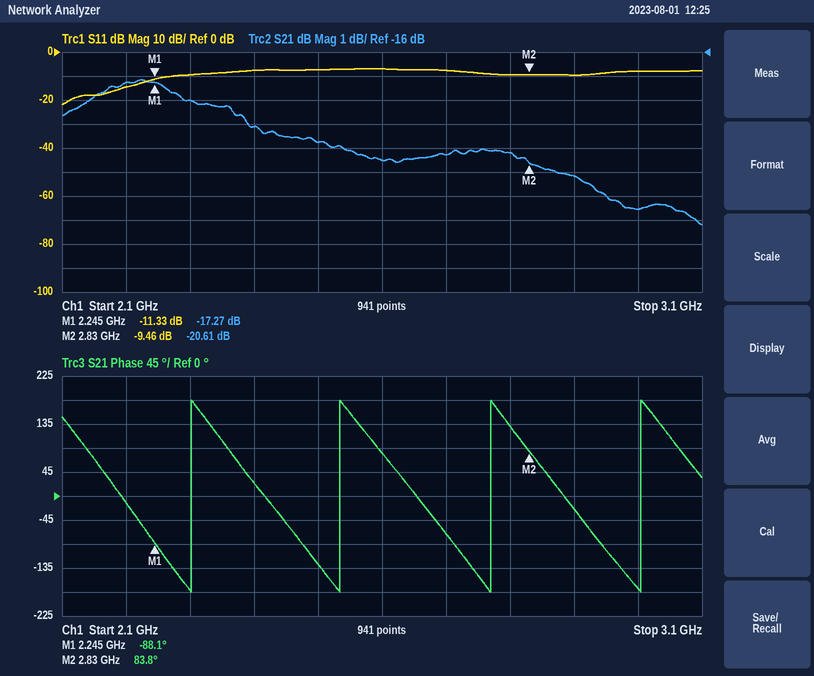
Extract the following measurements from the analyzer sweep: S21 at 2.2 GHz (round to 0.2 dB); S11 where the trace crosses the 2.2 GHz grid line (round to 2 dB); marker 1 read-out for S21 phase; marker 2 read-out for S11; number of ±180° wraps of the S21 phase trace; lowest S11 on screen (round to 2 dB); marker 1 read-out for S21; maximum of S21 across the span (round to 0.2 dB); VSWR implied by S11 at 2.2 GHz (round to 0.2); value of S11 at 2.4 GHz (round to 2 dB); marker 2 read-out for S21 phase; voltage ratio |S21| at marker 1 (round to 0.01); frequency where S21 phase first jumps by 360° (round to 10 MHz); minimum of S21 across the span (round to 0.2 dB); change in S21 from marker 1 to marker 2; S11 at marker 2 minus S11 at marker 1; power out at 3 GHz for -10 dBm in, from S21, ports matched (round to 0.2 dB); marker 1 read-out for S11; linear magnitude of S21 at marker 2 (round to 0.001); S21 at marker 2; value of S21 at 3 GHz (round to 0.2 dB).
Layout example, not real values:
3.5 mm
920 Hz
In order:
-17.2 dB
-14 dB
-88.1°
-9.46 dB
4
-22 dB
-17.27 dB
-17.2 dB
1.4
-8 dB
83.8°
0.14
2.30 GHz
-23.2 dB
-3.34 dB
1.87 dB
-32.6 dBm
-11.33 dB
0.093
-20.61 dB
-22.6 dB
